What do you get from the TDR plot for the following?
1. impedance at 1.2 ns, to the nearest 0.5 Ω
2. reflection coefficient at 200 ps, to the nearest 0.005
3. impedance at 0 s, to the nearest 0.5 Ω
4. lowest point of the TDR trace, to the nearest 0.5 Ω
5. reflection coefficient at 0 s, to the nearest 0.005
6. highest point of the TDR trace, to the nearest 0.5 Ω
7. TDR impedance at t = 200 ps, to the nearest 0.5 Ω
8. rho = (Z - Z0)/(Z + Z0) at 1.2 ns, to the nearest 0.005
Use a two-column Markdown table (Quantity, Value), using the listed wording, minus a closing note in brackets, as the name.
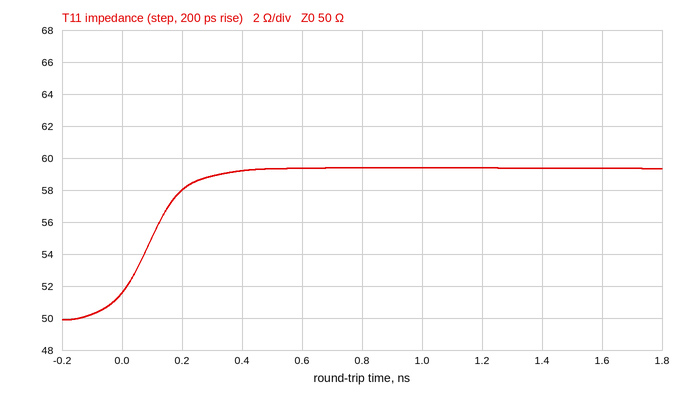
| Quantity | Value |
|---|---|
| impedance at 1.2 ns, to the nearest 0.5 Ω | 59.5 Ω |
| reflection coefficient at 200 ps, to the nearest 0.005 | +0.075 |
| impedance at 0 s, to the nearest 0.5 Ω | 51.5 Ω |
| lowest point of the TDR trace, to the nearest 0.5 Ω | 50.0 Ω |
| reflection coefficient at 0 s, to the nearest 0.005 | +0.015 |
| highest point of the TDR trace, to the nearest 0.5 Ω | 59.5 Ω |
| TDR impedance at t = 200 ps, to the nearest 0.5 Ω | 58.0 Ω |
| rho = (Z - Z0)/(Z + Z0) at 1.2 ns, to the nearest 0.005 | +0.085 |
